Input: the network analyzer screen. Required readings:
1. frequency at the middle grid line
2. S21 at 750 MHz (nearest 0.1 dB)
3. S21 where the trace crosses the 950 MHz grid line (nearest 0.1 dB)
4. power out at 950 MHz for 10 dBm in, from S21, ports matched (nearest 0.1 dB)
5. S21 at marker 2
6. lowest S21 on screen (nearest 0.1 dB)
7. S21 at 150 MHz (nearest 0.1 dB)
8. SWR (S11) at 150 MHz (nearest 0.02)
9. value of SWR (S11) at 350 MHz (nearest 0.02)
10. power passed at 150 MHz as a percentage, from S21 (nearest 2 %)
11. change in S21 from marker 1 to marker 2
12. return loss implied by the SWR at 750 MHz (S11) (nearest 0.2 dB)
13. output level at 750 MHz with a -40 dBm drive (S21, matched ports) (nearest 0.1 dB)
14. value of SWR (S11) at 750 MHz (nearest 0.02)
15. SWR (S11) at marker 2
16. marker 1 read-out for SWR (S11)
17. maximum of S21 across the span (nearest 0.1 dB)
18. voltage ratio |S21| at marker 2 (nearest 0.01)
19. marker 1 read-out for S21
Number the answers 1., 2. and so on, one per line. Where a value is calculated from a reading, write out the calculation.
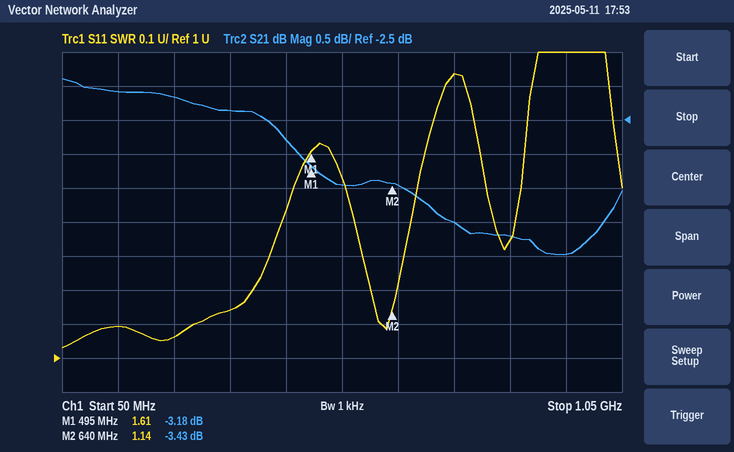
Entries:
1. 550 MHz
2. -4.0 dB
3. -4.5 dB
4. 10 dBm + (-4.5 dB) = 5.5 dBm
5. -3.43 dB
6. -4.5 dB
7. -2.1 dB
8. 1.10
9. 1.14
10. 10^(-2.1/10) ≈ 62 %
11. -3.43 − (-3.18) = -0.25 dB
12. −20 log10((1.84 − 1)/(1.84 + 1)) ≈ 10.6 dB
13. -40 dBm + (-4.0 dB) = -44.0 dBm
14. 1.84
15. 1.14
16. 1.61
17. -1.9 dB
18. 10^(-3.43/20) ≈ 0.67
19. -3.18 dB
